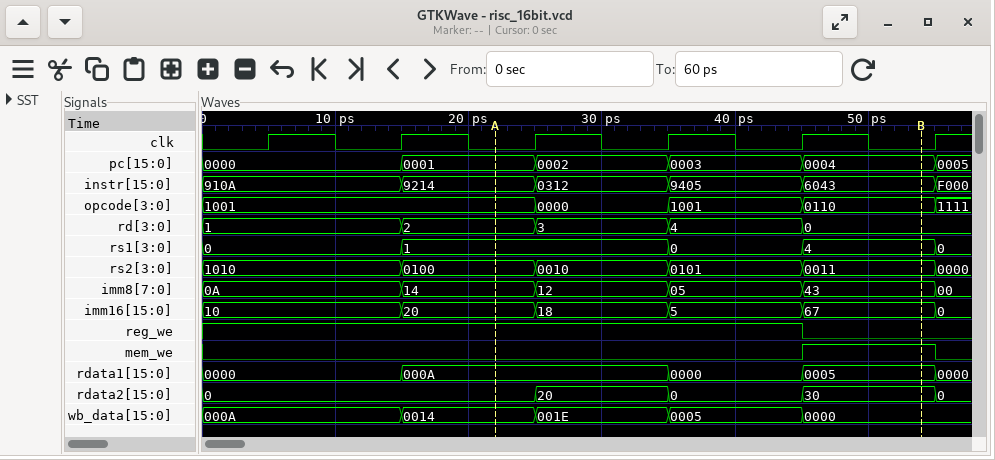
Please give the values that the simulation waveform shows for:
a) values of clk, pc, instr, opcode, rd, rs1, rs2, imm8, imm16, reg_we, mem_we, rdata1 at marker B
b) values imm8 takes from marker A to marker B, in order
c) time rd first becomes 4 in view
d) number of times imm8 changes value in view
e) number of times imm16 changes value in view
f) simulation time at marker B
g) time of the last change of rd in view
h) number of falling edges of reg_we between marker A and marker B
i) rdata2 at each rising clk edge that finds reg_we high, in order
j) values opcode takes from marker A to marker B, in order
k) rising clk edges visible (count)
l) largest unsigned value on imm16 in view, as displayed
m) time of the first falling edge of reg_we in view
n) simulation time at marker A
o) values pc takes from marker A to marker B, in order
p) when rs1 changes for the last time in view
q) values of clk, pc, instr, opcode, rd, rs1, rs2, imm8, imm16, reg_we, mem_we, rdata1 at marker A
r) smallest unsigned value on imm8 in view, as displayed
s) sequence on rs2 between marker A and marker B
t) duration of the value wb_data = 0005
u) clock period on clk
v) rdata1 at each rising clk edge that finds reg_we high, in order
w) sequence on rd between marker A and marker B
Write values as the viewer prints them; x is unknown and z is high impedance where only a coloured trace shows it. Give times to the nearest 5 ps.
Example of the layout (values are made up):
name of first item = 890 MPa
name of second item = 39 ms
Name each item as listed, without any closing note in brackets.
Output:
values of clk, pc, instr, opcode, rd, rs1, rs2, imm8, imm16, reg_we, mem_we, rdata1 at marker B = clk=0, pc=0004, instr=6043, opcode=0110, rd=0, rs1=4, rs2=0011, imm8=43, imm16=67, reg_we=0, mem_we=1, rdata1=0005
values imm8 takes from marker A to marker B, in order = 14, 12, 05, 43
time rd first becomes 4 in view = 35 ps
number of times imm8 changes value in view = 5
number of times imm16 changes value in view = 5
simulation time at marker B = 55 ps
time of the last change of rd in view = 45 ps
number of falling edges of reg_we between marker A and marker B = 1
rdata2 at each rising clk edge that finds reg_we high, in order = 0, 0, 0, 20, 0
values opcode takes from marker A to marker B, in order = 1001, 0000, 1001, 0110
rising clk edges visible = 6
largest unsigned value on imm16 in view, as displayed = 67
time of the first falling edge of reg_we in view = 45 ps
simulation time at marker A = 20 ps
values pc takes from marker A to marker B, in order = 0001, 0002, 0003, 0004
when rs1 changes for the last time in view = 55 ps
values of clk, pc, instr, opcode, rd, rs1, rs2, imm8, imm16, reg_we, mem_we, rdata1 at marker A = clk=0, pc=0001, instr=9214, opcode=1001, rd=2, rs1=1, rs2=0100, imm8=14, imm16=20, reg_we=1, mem_we=0, rdata1=000A
smallest unsigned value on imm8 in view, as displayed = 00
sequence on rs2 between marker A and marker B = 0100, 0010, 0101, 0011
duration of the value wb_data = 0005 = 10 ps
clock period on clk = 10 ps
rdata1 at each rising clk edge that finds reg_we high, in order = 0000, 0000, 000A, 000A, 0000
sequence on rd between marker A and marker B = 2, 3, 4, 0
